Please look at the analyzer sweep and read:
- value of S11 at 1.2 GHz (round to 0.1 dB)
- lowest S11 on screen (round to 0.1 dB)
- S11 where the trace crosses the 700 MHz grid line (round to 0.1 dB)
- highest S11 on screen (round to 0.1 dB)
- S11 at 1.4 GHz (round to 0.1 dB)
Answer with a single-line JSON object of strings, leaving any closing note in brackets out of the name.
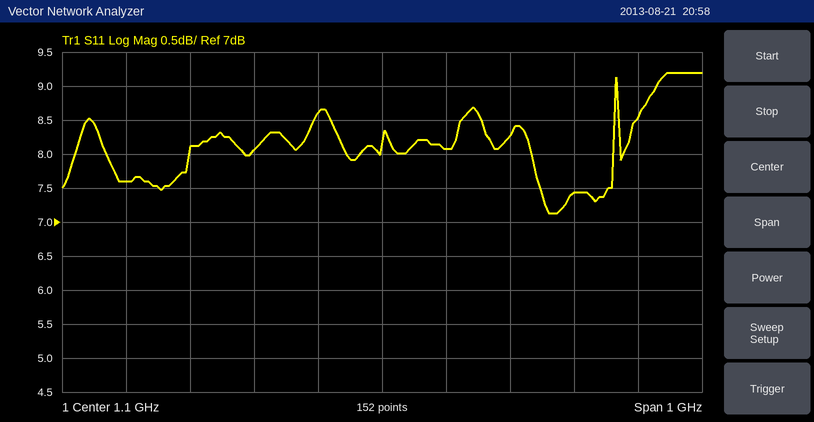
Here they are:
{"value of S11 at 1.2 GHz": "8.1 dB", "lowest S11 on screen": "7.1 dB", "S11 where the trace crosses the 700 MHz grid line": "7.6 dB", "highest S11 on screen": "9.2 dB", "S11 at 1.4 GHz": "7.4 dB"}
